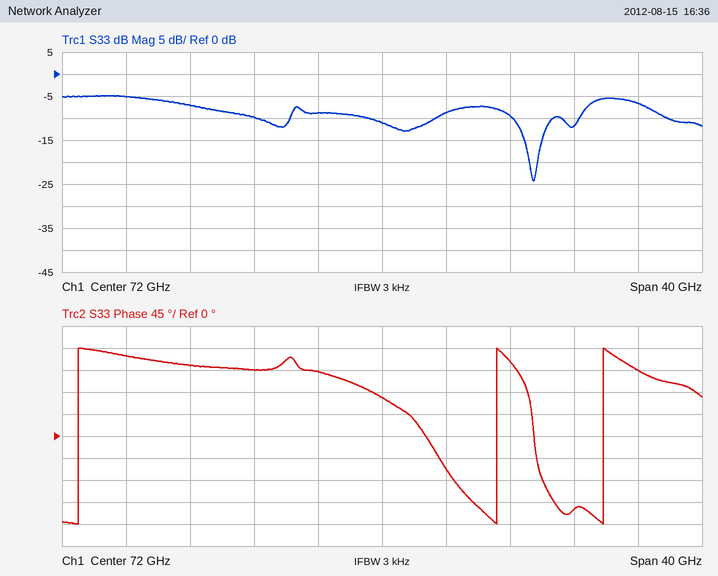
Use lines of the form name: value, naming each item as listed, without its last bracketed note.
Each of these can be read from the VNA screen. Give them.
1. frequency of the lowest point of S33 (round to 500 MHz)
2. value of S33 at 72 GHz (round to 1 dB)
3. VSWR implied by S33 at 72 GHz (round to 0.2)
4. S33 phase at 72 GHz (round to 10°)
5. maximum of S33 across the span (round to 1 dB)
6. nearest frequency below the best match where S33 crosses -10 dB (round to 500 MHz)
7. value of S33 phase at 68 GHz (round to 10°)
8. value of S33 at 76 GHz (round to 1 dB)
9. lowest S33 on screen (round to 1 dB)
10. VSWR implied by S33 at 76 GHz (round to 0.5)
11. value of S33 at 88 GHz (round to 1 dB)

frequency of the lowest point of S33: 81.5 GHz
value of S33 at 72 GHz: -11 dB
VSWR implied by S33 at 72 GHz: 1.8
S33 phase at 72 GHz: 80°
maximum of S33 across the span: -5 dB
nearest frequency below the best match where S33 crosses -10 dB: 80.0 GHz
value of S33 phase at 68 GHz: 130°
value of S33 at 76 GHz: -9 dB
lowest S33 on screen: -24 dB
VSWR implied by S33 at 76 GHz: 2.0
value of S33 at 88 GHz: -7 dB
